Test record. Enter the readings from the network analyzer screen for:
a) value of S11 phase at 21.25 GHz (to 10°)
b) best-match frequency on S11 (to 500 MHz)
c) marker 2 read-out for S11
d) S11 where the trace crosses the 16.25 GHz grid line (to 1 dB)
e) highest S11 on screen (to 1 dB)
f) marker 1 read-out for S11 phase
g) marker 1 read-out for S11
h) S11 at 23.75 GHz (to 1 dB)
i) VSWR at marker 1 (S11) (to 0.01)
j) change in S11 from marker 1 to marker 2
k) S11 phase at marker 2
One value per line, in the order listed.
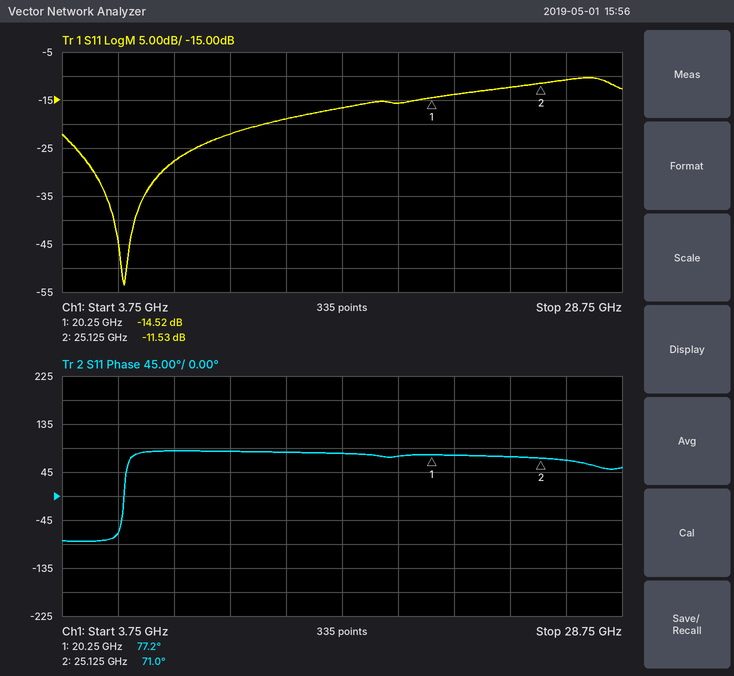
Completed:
80°
6.5 GHz
-11.53 dB
-17 dB
-10 dB
77.2°
-14.52 dB
-12 dB
1.46
2.99 dB
71.0°
